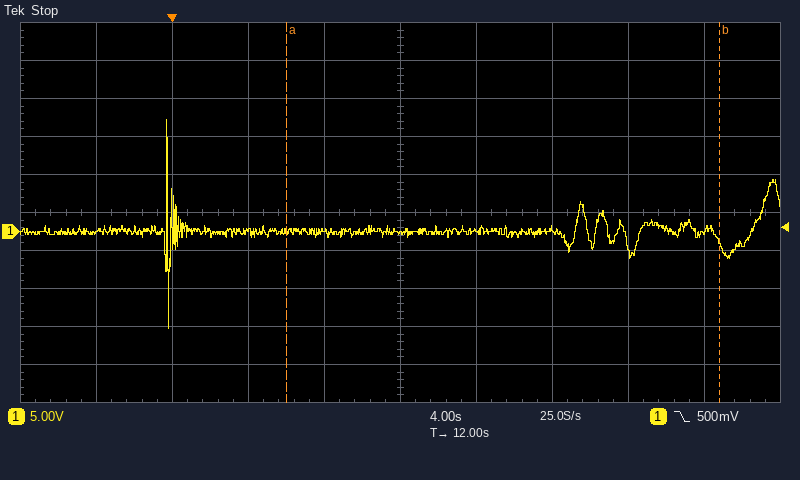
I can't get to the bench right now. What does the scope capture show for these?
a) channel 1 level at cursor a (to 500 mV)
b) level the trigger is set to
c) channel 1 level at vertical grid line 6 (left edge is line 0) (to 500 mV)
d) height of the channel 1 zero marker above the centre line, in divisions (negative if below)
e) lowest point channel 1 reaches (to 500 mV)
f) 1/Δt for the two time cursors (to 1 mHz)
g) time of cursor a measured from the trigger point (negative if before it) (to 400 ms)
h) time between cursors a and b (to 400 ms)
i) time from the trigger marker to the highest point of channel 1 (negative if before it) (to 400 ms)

0.0 V
500 mV
0.0 V
-0.5 div
-13.0 V
44 mHz
+6.0 s
22.8 s
-400 ms
